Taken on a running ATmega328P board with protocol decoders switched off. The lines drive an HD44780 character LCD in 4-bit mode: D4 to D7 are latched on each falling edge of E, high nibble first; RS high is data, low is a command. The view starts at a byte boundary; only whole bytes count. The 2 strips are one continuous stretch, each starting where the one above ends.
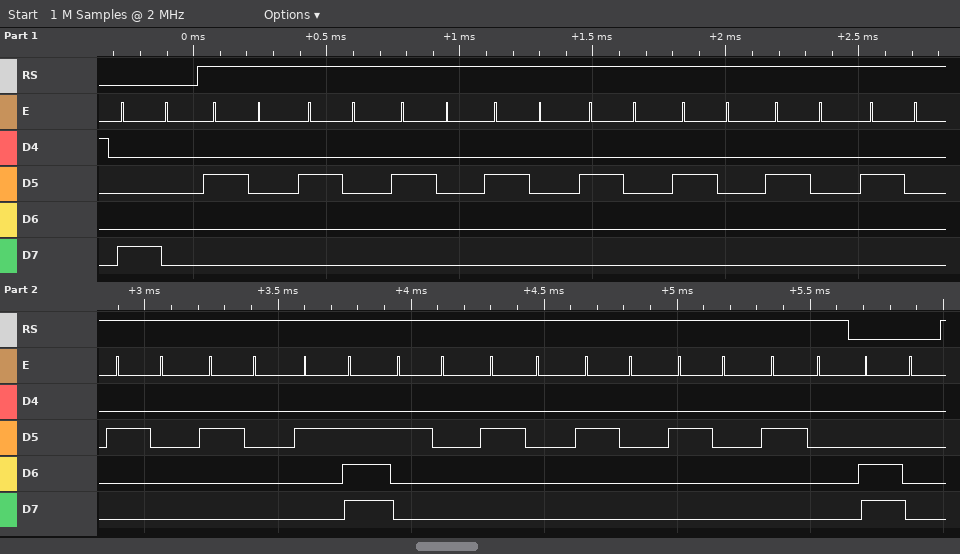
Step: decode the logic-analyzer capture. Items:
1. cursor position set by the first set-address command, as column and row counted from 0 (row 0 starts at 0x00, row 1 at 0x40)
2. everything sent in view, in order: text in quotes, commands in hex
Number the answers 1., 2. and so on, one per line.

1. column 0, row 0
2. 0x80 "          .     " 0xC0
